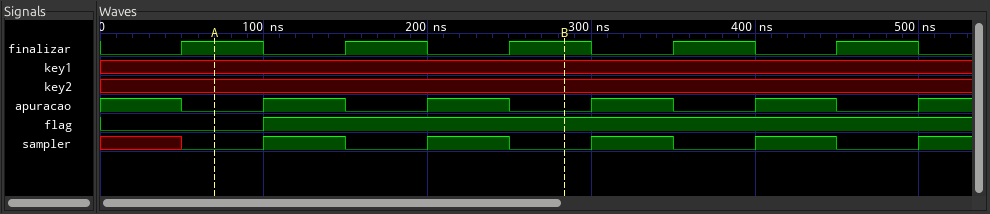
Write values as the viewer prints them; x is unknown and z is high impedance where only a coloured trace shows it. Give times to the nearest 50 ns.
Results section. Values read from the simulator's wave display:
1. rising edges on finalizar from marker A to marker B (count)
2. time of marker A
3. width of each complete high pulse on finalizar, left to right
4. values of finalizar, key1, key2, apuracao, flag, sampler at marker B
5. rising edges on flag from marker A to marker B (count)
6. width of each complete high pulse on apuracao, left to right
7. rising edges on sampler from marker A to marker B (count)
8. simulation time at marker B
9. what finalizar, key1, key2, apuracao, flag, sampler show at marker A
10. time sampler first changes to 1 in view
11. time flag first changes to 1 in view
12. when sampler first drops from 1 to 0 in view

2
50 ns
50 ns, 50 ns, 50 ns, 50 ns, 50 ns
finalizar=1, key1=x, key2=x, apuracao=0, flag=1, sampler=0
1
50 ns, 50 ns, 50 ns, 50 ns
2
300 ns
finalizar=1, key1=x, key2=x, apuracao=0, flag=0, sampler=0
100 ns
100 ns
150 ns
